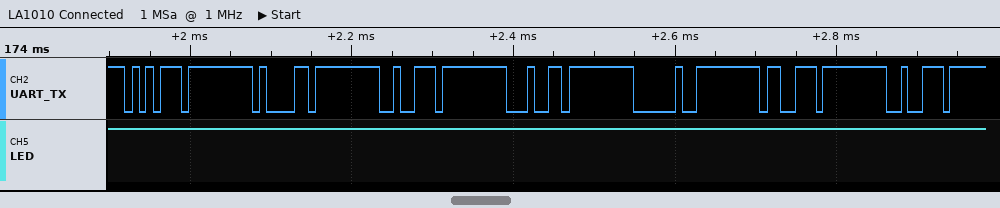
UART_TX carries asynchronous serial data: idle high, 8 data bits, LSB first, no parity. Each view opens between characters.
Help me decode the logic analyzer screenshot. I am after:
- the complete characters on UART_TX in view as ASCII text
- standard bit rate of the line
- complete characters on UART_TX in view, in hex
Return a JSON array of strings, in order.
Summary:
["\"uard sr\"", "115200 baud", "75, 61, 72, 64, 20, 73, 72"]
